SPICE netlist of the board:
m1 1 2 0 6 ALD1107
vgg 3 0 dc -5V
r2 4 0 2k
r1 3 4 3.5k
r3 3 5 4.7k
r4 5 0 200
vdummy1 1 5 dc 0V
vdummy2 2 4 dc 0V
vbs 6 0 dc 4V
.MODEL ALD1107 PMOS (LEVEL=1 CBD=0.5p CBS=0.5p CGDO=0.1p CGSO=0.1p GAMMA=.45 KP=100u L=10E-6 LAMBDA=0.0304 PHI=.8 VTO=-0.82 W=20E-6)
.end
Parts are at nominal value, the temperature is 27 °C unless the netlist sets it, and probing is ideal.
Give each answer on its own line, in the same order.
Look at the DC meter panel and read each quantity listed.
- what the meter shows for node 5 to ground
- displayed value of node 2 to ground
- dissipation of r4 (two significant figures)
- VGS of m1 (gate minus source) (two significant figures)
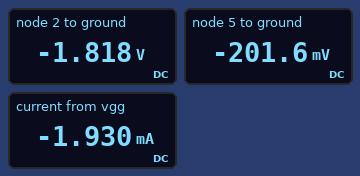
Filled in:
-201.6 mV
-1.818 V
200 µW
-1.8 V
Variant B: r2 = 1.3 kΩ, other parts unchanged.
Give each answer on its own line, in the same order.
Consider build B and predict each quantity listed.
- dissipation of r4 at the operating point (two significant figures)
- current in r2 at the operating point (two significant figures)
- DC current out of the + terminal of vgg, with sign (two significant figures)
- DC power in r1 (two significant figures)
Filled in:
210 µW
1.0 mA
-2.1 mA
3.8 mW
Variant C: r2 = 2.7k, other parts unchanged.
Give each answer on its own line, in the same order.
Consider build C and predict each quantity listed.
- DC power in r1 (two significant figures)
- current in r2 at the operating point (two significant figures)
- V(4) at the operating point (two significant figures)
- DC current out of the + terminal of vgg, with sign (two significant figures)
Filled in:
2.3 mW
810 µA
-2.2 V
-1.8 mA
